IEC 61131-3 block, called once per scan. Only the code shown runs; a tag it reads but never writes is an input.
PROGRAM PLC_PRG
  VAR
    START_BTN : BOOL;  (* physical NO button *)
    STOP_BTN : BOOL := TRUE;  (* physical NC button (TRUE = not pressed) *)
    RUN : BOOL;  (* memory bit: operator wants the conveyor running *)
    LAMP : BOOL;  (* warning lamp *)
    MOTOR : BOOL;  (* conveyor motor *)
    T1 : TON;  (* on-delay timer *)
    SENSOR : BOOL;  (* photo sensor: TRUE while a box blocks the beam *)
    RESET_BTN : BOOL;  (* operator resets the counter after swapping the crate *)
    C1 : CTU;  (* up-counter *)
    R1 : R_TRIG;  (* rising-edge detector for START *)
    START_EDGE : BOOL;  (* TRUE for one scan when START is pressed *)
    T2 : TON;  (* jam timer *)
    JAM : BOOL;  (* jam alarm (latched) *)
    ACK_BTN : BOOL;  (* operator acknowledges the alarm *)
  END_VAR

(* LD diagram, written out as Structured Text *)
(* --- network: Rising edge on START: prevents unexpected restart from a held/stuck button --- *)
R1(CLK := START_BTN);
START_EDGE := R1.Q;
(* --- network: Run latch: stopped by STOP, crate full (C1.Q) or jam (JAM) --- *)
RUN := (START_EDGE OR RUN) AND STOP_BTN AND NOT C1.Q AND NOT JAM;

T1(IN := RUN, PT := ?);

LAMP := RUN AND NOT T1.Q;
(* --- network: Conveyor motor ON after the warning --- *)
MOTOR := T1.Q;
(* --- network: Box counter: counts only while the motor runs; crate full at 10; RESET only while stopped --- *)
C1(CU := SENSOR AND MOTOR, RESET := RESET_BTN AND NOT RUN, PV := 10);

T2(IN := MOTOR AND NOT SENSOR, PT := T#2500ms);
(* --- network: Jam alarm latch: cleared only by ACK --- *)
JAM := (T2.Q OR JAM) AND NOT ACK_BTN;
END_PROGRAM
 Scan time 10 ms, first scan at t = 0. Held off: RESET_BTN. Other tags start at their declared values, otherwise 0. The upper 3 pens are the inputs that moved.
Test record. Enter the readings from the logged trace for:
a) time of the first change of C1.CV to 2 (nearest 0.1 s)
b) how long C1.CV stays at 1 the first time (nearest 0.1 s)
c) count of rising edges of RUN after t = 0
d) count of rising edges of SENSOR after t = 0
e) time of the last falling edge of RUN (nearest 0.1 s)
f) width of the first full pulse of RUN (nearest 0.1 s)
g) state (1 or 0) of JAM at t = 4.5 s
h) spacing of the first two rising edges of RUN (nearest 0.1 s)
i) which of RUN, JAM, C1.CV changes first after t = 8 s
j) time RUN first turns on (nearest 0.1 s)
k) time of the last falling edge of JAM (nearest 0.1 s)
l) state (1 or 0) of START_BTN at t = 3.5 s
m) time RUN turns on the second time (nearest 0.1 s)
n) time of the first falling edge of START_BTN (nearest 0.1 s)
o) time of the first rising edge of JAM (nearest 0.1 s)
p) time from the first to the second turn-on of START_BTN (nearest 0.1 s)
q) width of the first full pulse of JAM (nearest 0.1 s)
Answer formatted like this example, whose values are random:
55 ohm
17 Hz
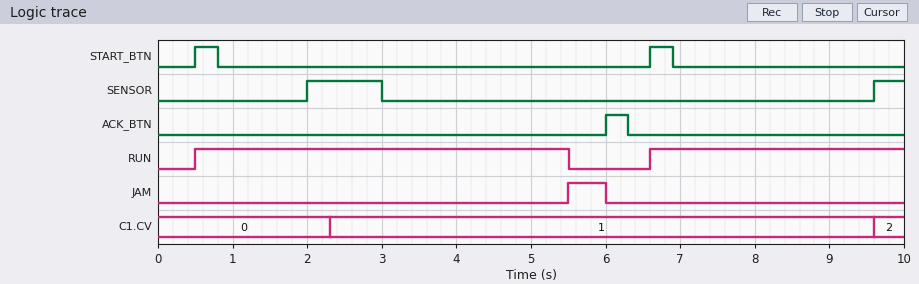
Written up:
9.6 s
7.3 s
2
2
5.5 s
5.0 s
0
6.1 s
C1.CV
0.5 s
6.0 s
0
6.6 s
0.8 s
5.5 s
6.1 s
0.5 s
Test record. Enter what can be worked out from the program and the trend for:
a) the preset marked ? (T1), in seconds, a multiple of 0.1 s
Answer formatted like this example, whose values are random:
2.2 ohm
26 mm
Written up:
1.8 s
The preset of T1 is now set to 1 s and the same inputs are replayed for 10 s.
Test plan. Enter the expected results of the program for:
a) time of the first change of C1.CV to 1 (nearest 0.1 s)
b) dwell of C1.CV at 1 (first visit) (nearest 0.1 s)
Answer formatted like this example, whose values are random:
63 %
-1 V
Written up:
2.0 s
7.6 s
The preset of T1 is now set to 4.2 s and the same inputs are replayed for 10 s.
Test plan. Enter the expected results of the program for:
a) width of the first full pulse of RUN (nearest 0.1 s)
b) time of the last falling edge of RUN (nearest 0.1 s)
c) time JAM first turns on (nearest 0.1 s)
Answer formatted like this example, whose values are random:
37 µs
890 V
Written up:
6.7 s
7.2 s
7.2 s
